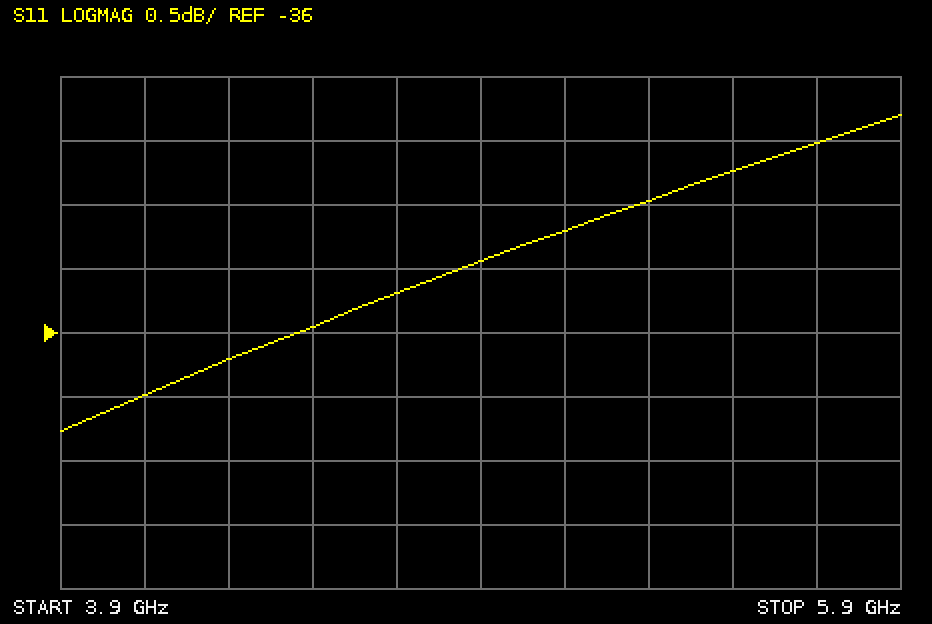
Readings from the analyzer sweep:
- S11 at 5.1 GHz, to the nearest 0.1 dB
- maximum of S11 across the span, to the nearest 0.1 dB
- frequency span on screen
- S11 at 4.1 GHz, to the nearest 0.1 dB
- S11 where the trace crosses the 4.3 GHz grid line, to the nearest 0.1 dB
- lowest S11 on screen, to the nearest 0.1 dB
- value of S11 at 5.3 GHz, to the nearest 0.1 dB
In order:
-35.2 dB
-34.3 dB
2 GHz
-36.5 dB
-36.2 dB
-36.8 dB
-35.0 dB
